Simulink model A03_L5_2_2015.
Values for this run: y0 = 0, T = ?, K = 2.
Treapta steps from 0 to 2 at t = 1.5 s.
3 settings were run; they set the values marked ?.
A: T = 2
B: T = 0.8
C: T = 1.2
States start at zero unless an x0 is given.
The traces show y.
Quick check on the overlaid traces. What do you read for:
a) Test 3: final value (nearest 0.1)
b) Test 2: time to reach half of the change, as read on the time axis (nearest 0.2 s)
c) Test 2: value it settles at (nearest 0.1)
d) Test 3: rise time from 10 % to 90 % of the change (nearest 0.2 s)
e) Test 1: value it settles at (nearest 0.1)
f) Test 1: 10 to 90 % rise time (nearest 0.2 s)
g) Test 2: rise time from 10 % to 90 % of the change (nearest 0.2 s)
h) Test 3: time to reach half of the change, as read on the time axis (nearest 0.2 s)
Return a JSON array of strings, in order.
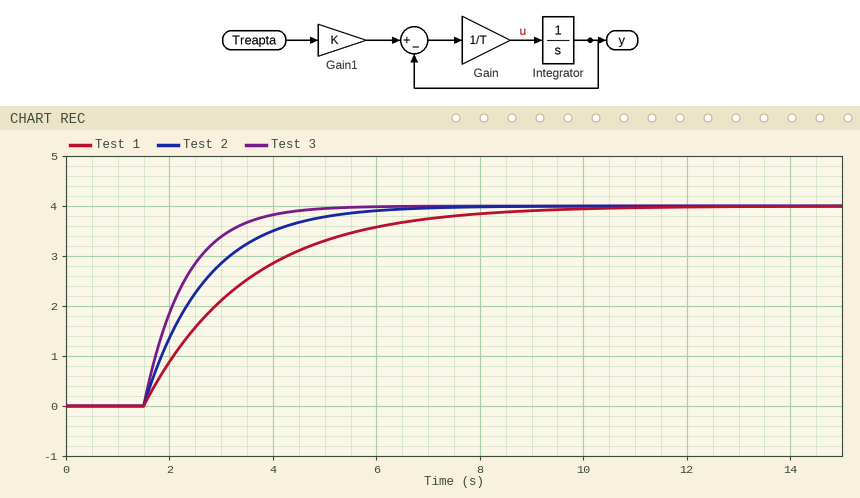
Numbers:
["4.0", "2.4 s", "4.0", "1.8 s", "4.0", "4.4 s", "2.6 s", "2.0 s"]
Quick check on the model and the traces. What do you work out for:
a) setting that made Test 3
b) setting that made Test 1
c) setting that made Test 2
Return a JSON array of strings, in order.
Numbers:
["B", "A", "C"]
